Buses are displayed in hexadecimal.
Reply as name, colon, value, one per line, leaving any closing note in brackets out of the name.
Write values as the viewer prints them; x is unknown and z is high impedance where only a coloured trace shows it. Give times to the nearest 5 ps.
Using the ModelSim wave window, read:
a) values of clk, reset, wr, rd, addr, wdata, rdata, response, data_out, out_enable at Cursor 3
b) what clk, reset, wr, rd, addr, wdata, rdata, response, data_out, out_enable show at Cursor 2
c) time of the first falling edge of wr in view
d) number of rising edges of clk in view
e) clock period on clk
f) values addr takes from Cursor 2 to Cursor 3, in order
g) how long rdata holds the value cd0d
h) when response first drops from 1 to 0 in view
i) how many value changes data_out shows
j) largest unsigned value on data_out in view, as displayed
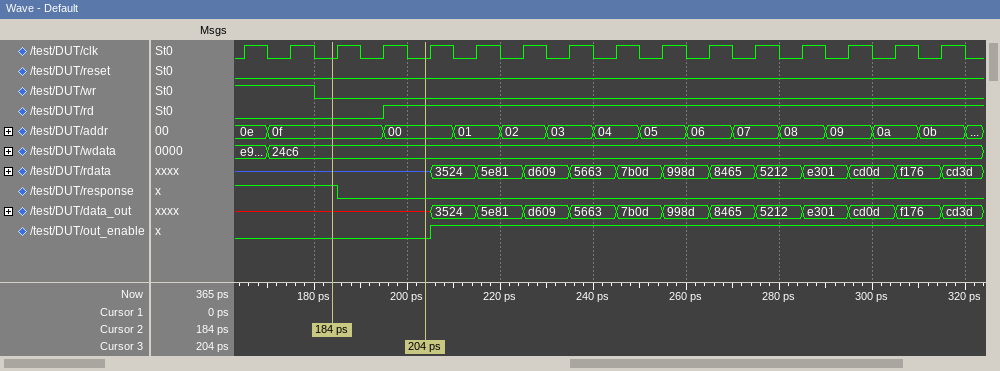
values of clk, reset, wr, rd, addr, wdata, rdata, response, data_out, out_enable at Cursor 3: clk=0, reset=0, wr=0, rd=1, addr=00, wdata=24c6, rdata=z, response=0, data_out=x, out_enable=0
what clk, reset, wr, rd, addr, wdata, rdata, response, data_out, out_enable show at Cursor 2: clk=0, reset=0, wr=0, rd=0, addr=0f, wdata=24c6, rdata=z, response=1, data_out=x, out_enable=0
time of the first falling edge of wr in view: 180 ps
number of rising edges of clk in view: 16
clock period on clk: 10 ps
values addr takes from Cursor 2 to Cursor 3, in order: 0f, 00
how long rdata holds the value cd0d: 10 ps
when response first drops from 1 to 0 in view: 185 ps
how many value changes data_out shows: 12
largest unsigned value on data_out in view, as displayed: f176
